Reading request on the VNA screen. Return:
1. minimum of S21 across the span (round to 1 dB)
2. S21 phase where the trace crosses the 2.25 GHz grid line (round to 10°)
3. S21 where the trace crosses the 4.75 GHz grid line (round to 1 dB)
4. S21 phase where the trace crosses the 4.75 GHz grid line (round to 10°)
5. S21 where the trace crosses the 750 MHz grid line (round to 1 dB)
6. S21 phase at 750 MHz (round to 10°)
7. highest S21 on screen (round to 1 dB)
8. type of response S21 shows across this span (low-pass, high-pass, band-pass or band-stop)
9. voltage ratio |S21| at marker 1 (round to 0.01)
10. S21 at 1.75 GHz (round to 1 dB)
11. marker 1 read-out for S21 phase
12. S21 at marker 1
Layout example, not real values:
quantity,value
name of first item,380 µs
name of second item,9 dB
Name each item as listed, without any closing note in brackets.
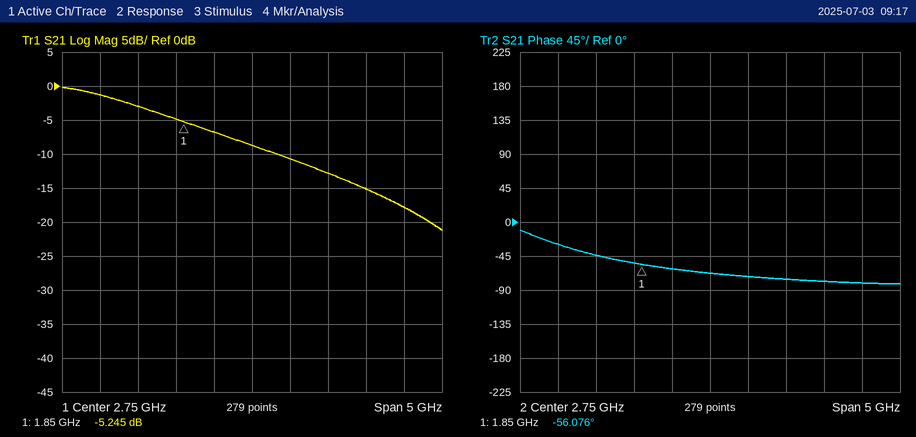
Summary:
quantity,value
minimum of S21 across the span,-21 dB
S21 phase where the trace crosses the 2.25 GHz grid line,-60°
S21 where the trace crosses the 4.75 GHz grid line,-18 dB
S21 phase where the trace crosses the 4.75 GHz grid line,-80°
S21 where the trace crosses the 750 MHz grid line,-1 dB
S21 phase at 750 MHz,-30°
highest S21 on screen,0 dB
type of response S21 shows across this span,low-pass
voltage ratio |S21| at marker 1,0.55
S21 at 1.75 GHz,-5 dB
marker 1 read-out for S21 phase,-56.076°
S21 at marker 1,-5.245 dB
